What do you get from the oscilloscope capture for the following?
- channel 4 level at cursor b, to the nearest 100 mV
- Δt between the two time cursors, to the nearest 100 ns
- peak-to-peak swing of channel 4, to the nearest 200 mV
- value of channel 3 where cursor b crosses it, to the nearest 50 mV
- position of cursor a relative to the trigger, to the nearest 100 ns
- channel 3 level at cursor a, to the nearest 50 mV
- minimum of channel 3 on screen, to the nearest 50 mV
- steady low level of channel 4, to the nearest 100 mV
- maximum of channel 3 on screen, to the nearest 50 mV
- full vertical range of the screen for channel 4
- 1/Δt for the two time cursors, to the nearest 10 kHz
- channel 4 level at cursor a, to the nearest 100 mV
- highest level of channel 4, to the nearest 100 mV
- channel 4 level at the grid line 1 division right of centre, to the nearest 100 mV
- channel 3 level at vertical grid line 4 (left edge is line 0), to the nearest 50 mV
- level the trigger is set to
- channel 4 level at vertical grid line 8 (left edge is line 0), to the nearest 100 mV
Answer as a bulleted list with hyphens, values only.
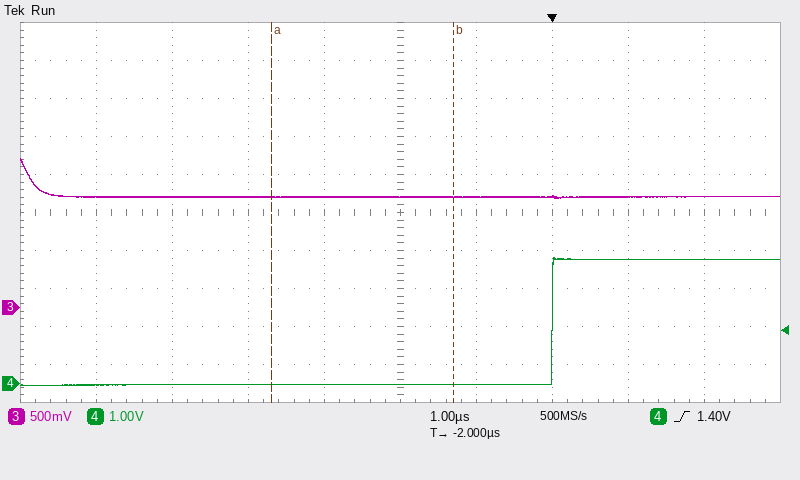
- 0.0 V
- 2.4 µs
- 3.4 V
- 1.45 V
- -3.7 µs
- 1.45 V
- 1.45 V
- 0.0 V
- 1.95 V
- 10 V
- 420 kHz
- 0.0 V
- 3.3 V
- 0.0 V
- 1.45 V
- 1.40 V
- 3.3 V
